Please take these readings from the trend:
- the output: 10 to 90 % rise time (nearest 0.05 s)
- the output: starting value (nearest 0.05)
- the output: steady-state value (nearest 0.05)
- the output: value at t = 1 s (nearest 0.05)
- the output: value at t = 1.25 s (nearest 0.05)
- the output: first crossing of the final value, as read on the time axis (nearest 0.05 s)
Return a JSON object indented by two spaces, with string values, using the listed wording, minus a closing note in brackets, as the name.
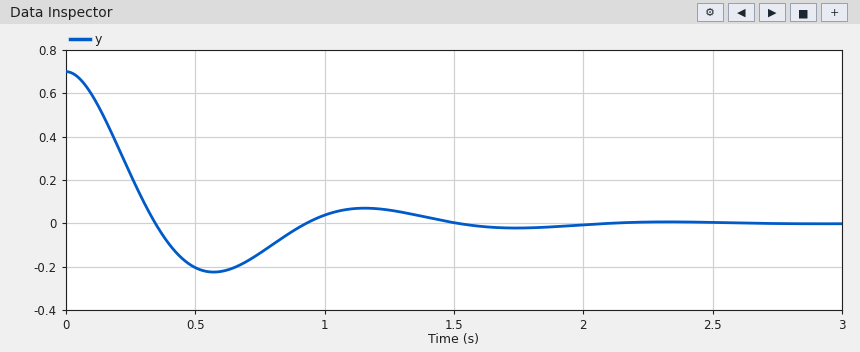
{
  "the output: 10 to 90 % rise time": "0.25 s",
  "the output: starting value": "0.70",
  "the output: steady-state value": "0.00",
  "the output: value at t = 1 s": "0.05",
  "the output: value at t = 1.25 s": "0.05",
  "the output: first crossing of the final value, as read on the time axis": "0.35 s"
}
